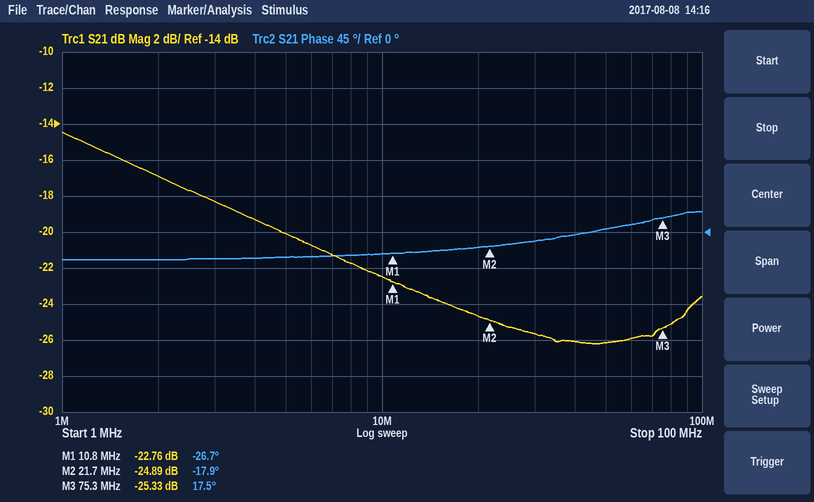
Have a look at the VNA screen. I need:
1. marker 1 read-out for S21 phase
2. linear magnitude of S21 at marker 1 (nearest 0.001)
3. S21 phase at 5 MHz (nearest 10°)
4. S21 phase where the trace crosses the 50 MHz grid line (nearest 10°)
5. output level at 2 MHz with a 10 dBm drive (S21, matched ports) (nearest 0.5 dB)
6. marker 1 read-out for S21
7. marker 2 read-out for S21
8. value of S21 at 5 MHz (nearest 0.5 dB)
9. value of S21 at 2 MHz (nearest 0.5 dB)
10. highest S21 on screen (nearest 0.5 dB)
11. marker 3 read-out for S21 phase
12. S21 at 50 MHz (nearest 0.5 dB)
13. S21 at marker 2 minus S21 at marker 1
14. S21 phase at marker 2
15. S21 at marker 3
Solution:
-26.7°
0.073
-30°
0°
-7.0 dBm
-22.76 dB
-24.89 dB
-20.0 dB
-17.0 dB
-14.5 dB
17.5°
-26.0 dB
-2.13 dB
-17.9°
-25.33 dB
